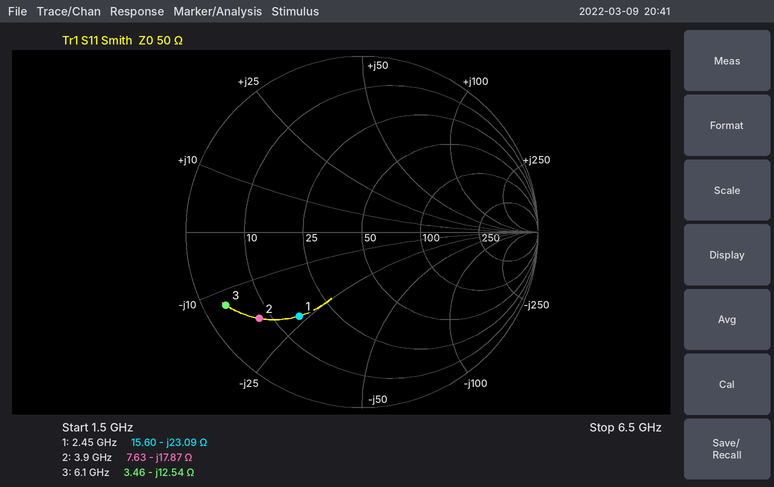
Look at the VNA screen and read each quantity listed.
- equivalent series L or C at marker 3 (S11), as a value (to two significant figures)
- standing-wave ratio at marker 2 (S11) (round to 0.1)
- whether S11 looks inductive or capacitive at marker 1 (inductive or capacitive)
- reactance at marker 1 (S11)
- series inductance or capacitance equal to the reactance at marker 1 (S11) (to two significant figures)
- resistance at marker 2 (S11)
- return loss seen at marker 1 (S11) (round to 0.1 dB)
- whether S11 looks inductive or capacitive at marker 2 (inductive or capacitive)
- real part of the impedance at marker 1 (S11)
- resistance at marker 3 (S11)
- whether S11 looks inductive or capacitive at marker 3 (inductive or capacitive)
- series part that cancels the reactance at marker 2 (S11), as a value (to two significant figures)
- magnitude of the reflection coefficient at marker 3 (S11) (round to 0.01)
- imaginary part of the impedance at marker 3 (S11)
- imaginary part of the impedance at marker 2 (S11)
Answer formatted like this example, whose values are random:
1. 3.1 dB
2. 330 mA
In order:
1. 2.1 pF
2. 7.4
3. capacitive
4. -23.09 Ω
5. 2.8 pF
6. 7.63 Ω
7. 4.5 dB
8. capacitive
9. 15.60 Ω
10. 3.46 Ω
11. capacitive
12. 730 pH
13. 0.88
14. -12.54 Ω
15. -17.87 Ω
